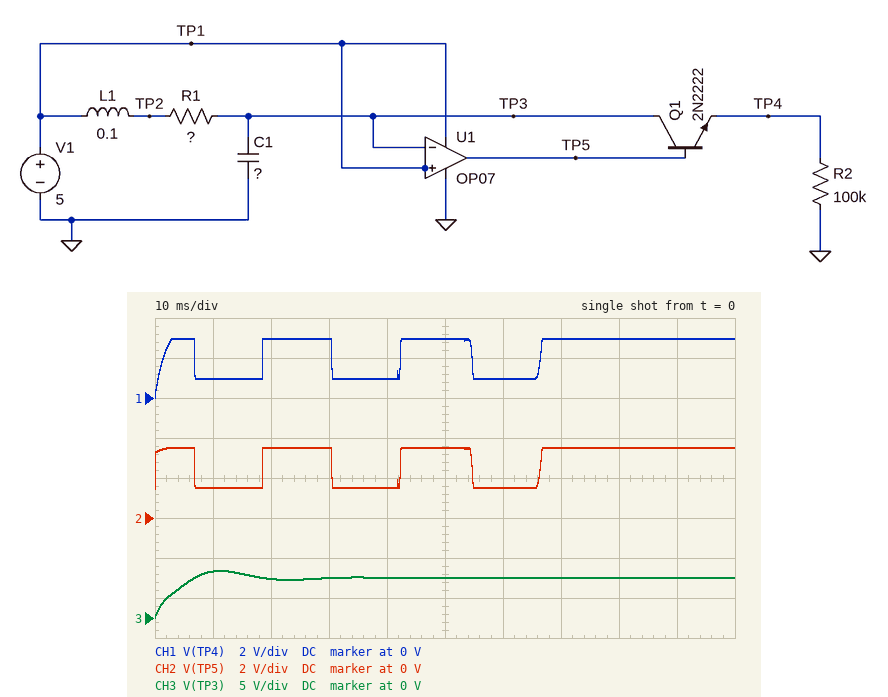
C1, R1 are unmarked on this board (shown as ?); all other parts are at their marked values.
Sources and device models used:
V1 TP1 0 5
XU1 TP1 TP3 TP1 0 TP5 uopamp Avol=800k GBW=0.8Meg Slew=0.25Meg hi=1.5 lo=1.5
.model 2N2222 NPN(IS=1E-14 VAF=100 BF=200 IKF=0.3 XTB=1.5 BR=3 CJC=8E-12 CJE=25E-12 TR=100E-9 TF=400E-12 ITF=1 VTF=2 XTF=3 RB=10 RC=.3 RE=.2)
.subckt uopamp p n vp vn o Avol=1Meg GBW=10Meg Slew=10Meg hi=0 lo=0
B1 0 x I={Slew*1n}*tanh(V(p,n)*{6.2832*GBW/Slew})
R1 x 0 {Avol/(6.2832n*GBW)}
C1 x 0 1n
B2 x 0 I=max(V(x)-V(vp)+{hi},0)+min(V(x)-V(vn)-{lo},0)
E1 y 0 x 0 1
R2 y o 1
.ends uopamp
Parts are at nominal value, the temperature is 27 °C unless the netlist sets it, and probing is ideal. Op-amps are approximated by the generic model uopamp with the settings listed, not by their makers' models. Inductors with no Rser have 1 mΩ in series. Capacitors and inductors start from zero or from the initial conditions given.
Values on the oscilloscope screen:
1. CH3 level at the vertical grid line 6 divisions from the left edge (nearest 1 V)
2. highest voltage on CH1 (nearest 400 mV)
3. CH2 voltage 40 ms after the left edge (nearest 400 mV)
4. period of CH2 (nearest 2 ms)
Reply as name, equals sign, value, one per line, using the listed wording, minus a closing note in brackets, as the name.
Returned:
CH3 level at the vertical grid line 6 divisions from the left edge = 5 V
highest voltage on CH1 = 2.8 V
CH2 voltage 40 ms after the left edge = 1.6 V
period of CH2 = 24 ms
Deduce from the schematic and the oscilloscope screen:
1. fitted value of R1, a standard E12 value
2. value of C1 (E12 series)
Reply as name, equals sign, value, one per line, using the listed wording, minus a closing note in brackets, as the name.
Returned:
fitted value of R1, a standard E12 value = 22 Ω
value of C1 = 120 µF
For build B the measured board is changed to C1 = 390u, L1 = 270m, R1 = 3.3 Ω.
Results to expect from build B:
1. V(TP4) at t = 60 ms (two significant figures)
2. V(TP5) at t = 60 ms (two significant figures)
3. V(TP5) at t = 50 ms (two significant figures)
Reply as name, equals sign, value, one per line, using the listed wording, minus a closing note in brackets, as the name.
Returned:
V(TP4) at t = 60 ms = 2.9 V
V(TP5) at t = 60 ms = 3.5 V
V(TP5) at t = 50 ms = 3.5 V
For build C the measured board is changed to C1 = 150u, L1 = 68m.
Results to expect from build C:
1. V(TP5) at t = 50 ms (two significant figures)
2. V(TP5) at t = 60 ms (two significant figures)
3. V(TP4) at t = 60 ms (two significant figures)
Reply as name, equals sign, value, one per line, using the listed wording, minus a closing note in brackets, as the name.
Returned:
V(TP5) at t = 50 ms = 3.5 V
V(TP5) at t = 60 ms = 3.5 V
V(TP4) at t = 60 ms = 2.9 V
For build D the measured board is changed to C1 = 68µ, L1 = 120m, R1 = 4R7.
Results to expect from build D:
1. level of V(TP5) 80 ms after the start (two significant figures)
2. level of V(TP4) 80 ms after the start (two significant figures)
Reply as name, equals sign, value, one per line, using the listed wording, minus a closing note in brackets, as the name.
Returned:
level of V(TP5) 80 ms after the start = 1.5 V
level of V(TP4) 80 ms after the start = 970 mV
